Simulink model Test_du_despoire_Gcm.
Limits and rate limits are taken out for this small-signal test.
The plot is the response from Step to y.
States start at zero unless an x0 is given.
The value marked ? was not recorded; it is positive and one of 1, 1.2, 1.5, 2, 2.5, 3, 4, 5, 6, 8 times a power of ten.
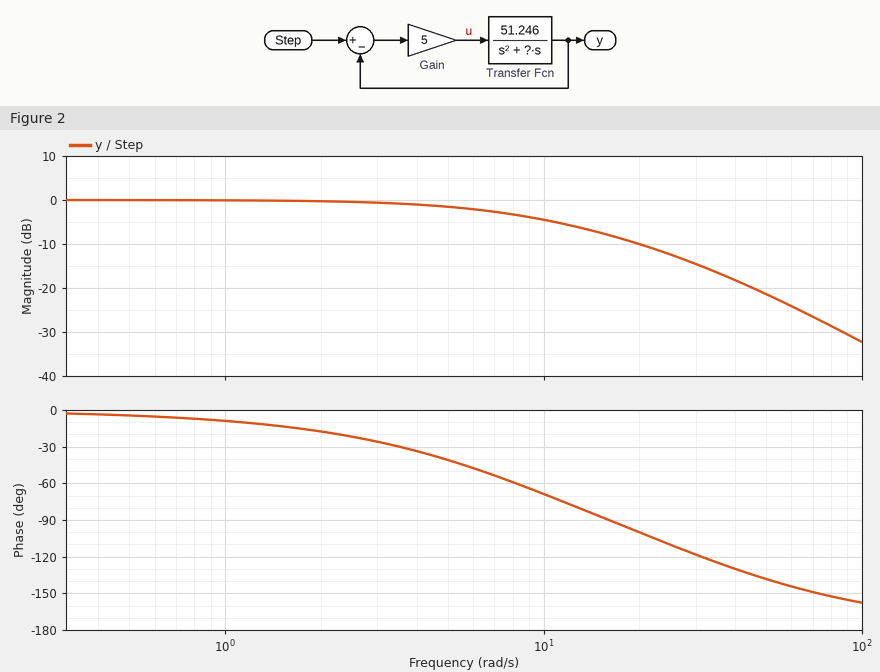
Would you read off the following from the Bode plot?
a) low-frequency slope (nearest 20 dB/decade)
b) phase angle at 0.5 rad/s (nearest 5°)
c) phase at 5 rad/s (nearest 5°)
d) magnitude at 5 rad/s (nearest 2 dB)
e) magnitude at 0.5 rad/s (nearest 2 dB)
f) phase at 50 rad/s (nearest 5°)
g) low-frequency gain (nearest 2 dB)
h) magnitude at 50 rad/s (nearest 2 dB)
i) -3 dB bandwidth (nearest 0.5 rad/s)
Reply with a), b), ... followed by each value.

a) 0 dB/decade
b) -5°
c) -40°
d) -2 dB
e) 0 dB
f) -140°
g) 0 dB
h) -22 dB
i) 7.5 rad/s
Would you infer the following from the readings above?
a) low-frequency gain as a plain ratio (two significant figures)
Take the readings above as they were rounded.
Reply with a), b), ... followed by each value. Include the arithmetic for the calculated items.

a) 10^(0 / 20) = 1.0
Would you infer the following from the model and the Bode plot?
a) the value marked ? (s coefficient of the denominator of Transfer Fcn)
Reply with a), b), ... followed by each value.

a) 40
